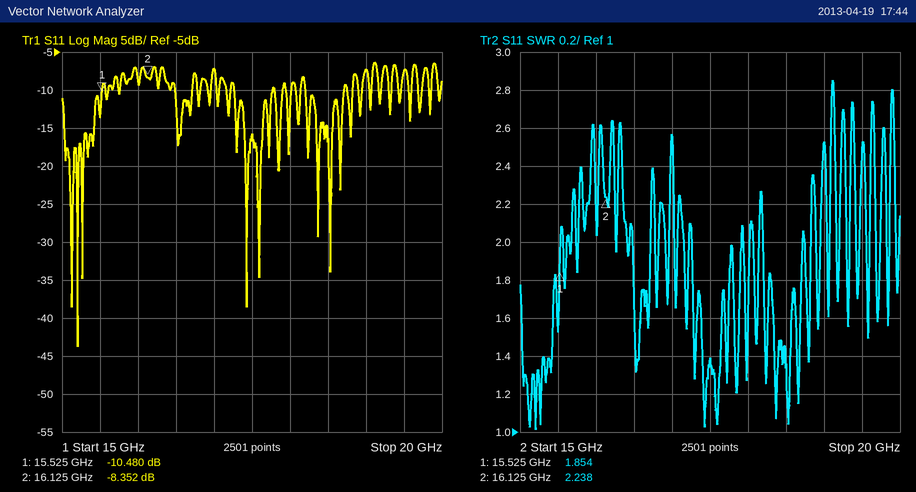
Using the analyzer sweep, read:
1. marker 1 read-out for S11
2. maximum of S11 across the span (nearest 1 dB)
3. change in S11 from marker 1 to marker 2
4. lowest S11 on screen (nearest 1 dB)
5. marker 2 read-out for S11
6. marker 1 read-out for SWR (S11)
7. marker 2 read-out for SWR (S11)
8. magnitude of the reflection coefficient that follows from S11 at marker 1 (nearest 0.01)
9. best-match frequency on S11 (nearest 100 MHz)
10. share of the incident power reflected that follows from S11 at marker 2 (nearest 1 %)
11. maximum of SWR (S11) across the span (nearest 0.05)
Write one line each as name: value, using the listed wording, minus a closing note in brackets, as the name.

marker 1 read-out for S11: -10.480 dB
maximum of S11 across the span: -6 dB
change in S11 from marker 1 to marker 2: 2.128 dB
lowest S11 on screen: -44 dB
marker 2 read-out for S11: -8.352 dB
marker 1 read-out for SWR: 1.854
marker 2 read-out for SWR: 2.238
magnitude of the reflection coefficient that follows from S11 at marker 1: 0.30
best-match frequency on S11: 15.2 GHz
share of the incident power reflected that follows from S11 at marker 2: 15 %
maximum of SWR (S11) across the span: 2.85
